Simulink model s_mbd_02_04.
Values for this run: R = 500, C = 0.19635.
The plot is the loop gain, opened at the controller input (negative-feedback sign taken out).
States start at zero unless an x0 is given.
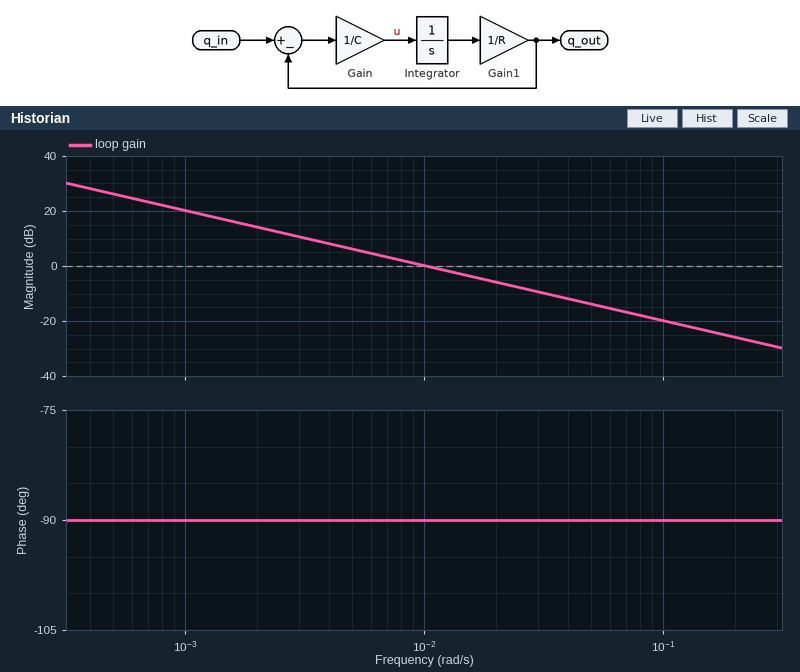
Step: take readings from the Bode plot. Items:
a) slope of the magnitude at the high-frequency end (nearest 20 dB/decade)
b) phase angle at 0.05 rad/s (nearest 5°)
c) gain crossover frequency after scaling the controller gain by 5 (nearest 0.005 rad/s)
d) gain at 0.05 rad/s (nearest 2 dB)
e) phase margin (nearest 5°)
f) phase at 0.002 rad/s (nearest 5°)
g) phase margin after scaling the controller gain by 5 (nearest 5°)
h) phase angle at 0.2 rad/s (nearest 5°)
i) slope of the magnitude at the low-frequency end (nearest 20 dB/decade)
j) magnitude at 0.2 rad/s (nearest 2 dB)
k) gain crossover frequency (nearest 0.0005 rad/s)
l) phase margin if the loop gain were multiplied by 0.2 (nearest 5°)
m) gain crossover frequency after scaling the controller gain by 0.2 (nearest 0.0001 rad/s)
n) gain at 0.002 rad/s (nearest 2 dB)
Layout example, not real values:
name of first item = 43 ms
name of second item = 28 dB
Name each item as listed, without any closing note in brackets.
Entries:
slope of the magnitude at the high-frequency end = -20 dB/decade
phase angle at 0.05 rad/s = -90°
gain crossover frequency after scaling the controller gain by 5 = 0.050 rad/s
gain at 0.05 rad/s = -14 dB
phase margin = 90°
phase at 0.002 rad/s = -90°
phase margin after scaling the controller gain by 5 = 90°
phase angle at 0.2 rad/s = -90°
slope of the magnitude at the low-frequency end = -20 dB/decade
magnitude at 0.2 rad/s = -26 dB
gain crossover frequency = 0.0100 rad/s
phase margin if the loop gain were multiplied by 0.2 = 90°
gain crossover frequency after scaling the controller gain by 0.2 = 0.0020 rad/s
gain at 0.002 rad/s = 14 dB
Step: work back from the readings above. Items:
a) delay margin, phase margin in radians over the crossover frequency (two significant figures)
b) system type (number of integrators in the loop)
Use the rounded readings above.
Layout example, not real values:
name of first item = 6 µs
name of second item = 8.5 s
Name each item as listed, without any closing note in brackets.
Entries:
delay margin, phase margin in radians over the crossover frequency = 160 s
system type = 1
